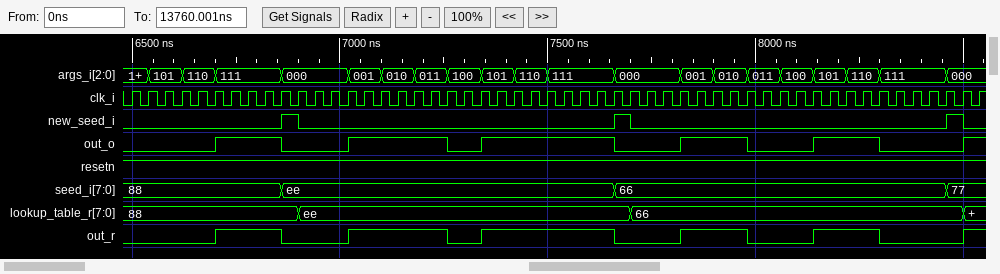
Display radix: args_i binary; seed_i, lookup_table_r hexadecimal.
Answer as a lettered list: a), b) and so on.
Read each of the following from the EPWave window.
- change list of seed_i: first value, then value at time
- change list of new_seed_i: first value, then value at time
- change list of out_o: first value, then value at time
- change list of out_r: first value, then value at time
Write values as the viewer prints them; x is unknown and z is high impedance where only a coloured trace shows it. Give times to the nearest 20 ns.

a) 88, ee at 6860 ns, 66 at 7660 ns, 77 at 8460 ns
b) 0, 1 at 6860 ns, 0 at 6900 ns, 1 at 7660 ns, 0 at 7700 ns, 1 at 8460 ns, 0 at 8500 ns
c) 0, 1 at 6700 ns, 0 at 6860 ns, 1 at 7020 ns, 0 at 7260 ns, 1 at 7340 ns, 0 at 7660 ns, 1 at 7820 ns, 0 at 7980 ns, 1 at 8140 ns, 0 at 8300 ns, 1 at 8500 ns
d) 0, 1 at 6700 ns, 0 at 6860 ns, 1 at 7020 ns, 0 at 7260 ns, 1 at 7340 ns, 0 at 7660 ns, 1 at 7820 ns, 0 at 7980 ns, 1 at 8140 ns, 0 at 8300 ns, 1 at 8500 ns
